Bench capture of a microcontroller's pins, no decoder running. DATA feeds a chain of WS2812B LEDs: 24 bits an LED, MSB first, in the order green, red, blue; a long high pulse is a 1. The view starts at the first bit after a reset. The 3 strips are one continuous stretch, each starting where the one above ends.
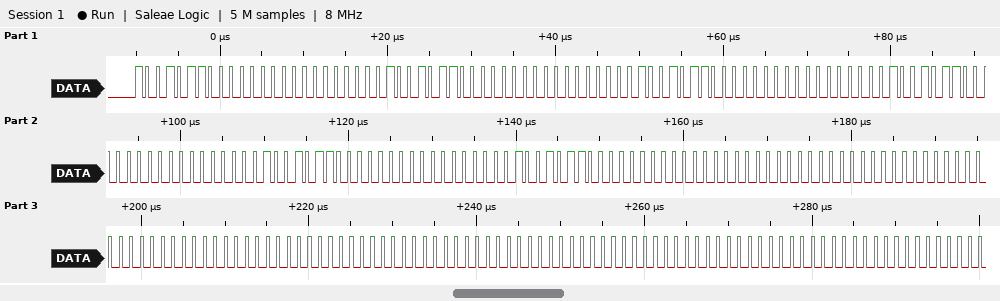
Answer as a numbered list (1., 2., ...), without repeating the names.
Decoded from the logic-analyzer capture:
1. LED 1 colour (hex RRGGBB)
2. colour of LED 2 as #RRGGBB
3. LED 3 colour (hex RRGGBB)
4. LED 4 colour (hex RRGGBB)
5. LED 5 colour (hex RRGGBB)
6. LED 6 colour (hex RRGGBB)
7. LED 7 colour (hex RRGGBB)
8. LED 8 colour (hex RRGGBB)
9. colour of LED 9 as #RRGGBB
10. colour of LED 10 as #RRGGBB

1. #009600
2. #009600
3. #009600
4. #009600
5. #009600
6. #009600
7. #000000
8. #000000
9. #000000
10. #000000
